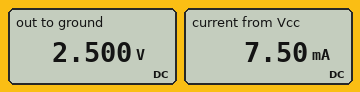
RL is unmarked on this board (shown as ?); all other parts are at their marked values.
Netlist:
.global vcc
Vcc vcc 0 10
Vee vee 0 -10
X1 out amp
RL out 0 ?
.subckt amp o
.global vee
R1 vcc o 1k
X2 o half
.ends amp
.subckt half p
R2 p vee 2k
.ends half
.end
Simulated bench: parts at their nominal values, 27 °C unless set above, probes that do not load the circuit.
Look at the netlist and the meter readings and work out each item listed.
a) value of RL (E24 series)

2 kΩ
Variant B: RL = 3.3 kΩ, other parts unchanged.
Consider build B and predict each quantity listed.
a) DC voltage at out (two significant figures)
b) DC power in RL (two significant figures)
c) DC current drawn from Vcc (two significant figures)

2.8 V
2.3 mW
7.2 mA
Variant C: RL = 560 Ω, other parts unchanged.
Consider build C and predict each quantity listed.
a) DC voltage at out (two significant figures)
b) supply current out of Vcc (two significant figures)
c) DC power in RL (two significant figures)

1.5 V
8.5 mA
4.1 mW
